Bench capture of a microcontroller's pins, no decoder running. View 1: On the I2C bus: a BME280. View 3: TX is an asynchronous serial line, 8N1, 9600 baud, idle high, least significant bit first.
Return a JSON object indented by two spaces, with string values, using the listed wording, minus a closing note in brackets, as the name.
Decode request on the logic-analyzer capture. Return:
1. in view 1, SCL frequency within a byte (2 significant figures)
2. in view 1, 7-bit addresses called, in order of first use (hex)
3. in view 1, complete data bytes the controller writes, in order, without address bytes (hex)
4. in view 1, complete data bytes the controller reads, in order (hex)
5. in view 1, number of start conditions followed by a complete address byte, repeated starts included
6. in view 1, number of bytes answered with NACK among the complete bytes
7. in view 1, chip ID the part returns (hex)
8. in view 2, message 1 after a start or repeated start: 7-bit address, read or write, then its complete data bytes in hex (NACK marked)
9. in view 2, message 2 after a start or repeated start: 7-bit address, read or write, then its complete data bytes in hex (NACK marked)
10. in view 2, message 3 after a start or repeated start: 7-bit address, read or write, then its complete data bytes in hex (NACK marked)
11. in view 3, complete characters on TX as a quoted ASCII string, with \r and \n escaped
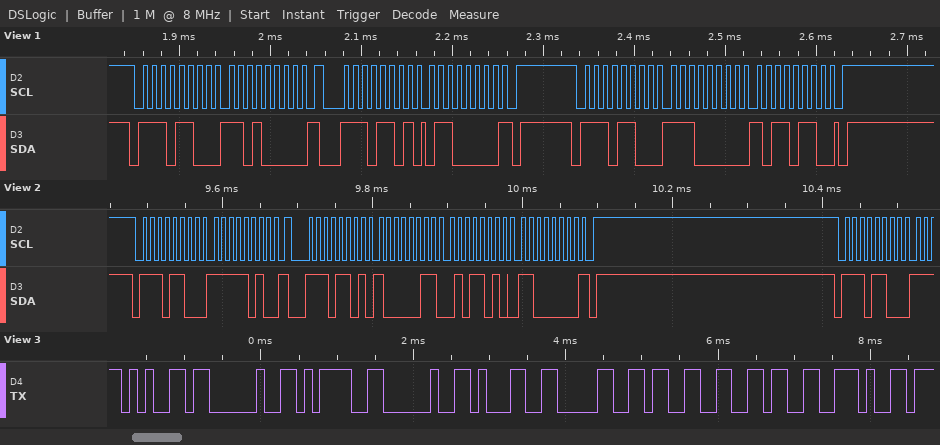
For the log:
{
  "in view 1, SCL frequency within a byte": "100 kHz",
  "in view 1, 7-bit addresses called, in order of first use": "0x76",
  "in view 1, complete data bytes the controller writes, in order, without address bytes": "D0 E0 B6",
  "in view 1, complete data bytes the controller reads, in order": "60",
  "in view 1, number of start conditions followed by a complete address byte, repeated starts included": "3",
  "in view 1, number of bytes answered with NACK among the complete bytes": "1",
  "in view 1, chip ID the part returns": "0x60",
  "in view 2, message 1 after a start or repeated start: 7-bit address, read or write, then its complete data bytes in hex": "0x76 write: FA",
  "in view 2, message 2 after a start or repeated start: 7-bit address, read or write, then its complete data bytes in hex": "0x76 read: 83 5A C0 NACK",
  "in view 2, message 3 after a start or repeated start: 7-bit address, read or write, then its complete data bytes in hex": "0x76 write",
  "in view 3, complete characters on TX as a quoted ASCII string, with \\r and \\n escaped": "\"e = 1036.\""
}
